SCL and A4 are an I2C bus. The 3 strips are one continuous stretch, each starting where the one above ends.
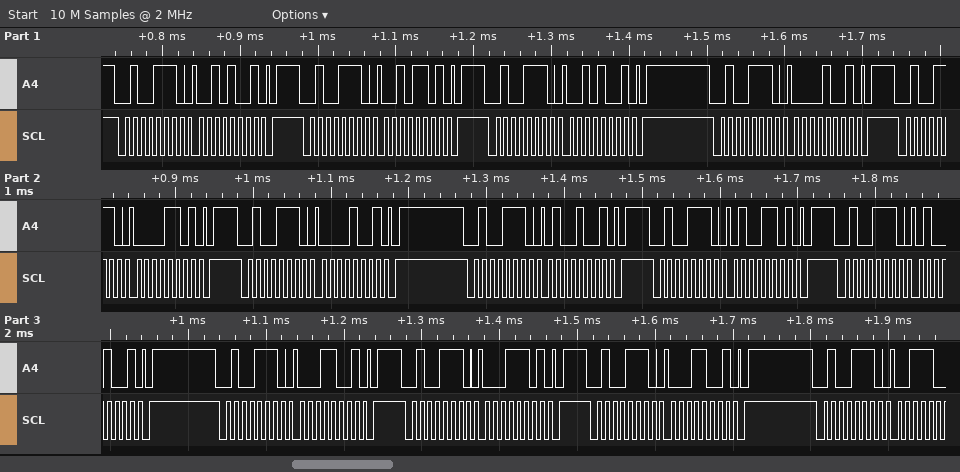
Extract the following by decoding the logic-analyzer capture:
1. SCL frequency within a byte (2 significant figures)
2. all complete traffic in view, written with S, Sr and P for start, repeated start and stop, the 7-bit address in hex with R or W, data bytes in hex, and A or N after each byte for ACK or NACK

100 kHz
S 27W A 29 A P S 27W A 2D A P S 27W A 29 A P S 27W A 09 A P S 27W A 0D A P S 27W A 09 A P S 27W A 49 A P S 27W A 4D A P S 27W A 49 A P S 27W A 19 A P S 27W A 1D A P S 27W A 19 A P S 27W A
